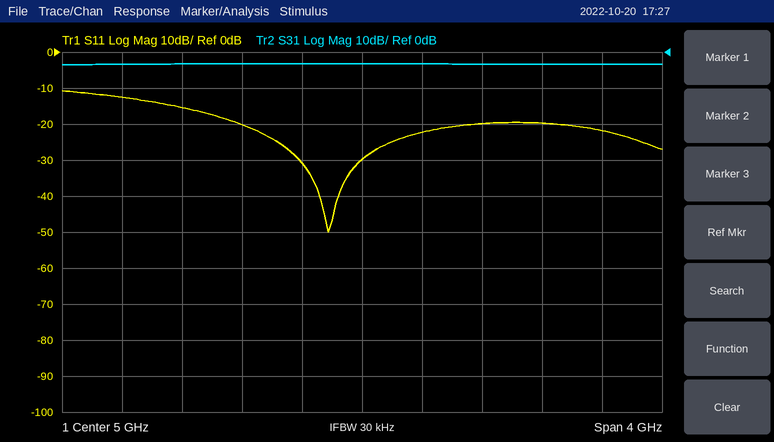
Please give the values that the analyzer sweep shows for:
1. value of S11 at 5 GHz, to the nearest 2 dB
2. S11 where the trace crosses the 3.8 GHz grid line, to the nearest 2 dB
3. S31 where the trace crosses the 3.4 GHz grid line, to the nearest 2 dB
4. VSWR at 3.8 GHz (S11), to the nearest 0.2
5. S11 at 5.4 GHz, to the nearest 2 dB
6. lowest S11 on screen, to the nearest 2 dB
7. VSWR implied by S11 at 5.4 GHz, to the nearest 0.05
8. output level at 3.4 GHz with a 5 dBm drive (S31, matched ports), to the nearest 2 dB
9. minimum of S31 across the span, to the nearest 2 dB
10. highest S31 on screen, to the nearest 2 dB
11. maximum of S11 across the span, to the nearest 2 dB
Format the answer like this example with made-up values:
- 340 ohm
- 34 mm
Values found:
- -30 dB
- -16 dB
- -4 dB
- 1.4
- -22 dB
- -50 dB
- 1.15
- 2 dBm
- -4 dB
- -4 dB
- -10 dB
